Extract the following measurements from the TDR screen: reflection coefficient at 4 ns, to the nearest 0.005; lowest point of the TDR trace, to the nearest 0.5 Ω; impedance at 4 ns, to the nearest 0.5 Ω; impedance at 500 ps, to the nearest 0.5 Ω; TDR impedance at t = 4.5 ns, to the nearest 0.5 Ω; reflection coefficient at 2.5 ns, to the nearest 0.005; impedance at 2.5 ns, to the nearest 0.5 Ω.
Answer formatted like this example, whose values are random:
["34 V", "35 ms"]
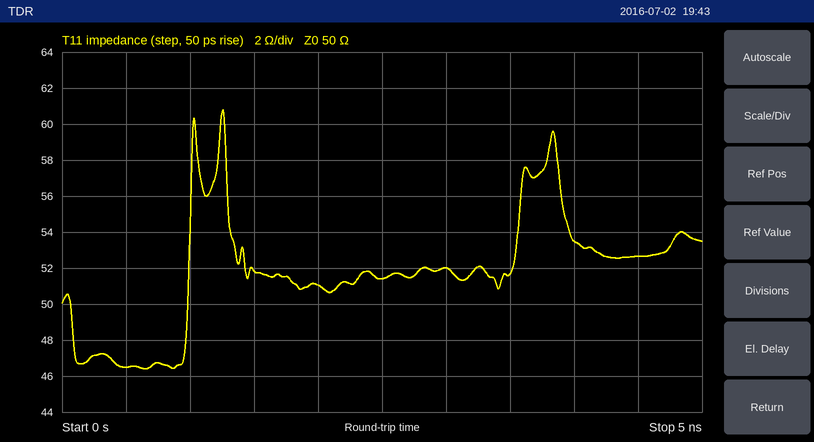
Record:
["+0.035", "46.5 Ω", "53.5 Ω", "46.5 Ω", "52.5 Ω", "+0.015", "51.5 Ω"]
